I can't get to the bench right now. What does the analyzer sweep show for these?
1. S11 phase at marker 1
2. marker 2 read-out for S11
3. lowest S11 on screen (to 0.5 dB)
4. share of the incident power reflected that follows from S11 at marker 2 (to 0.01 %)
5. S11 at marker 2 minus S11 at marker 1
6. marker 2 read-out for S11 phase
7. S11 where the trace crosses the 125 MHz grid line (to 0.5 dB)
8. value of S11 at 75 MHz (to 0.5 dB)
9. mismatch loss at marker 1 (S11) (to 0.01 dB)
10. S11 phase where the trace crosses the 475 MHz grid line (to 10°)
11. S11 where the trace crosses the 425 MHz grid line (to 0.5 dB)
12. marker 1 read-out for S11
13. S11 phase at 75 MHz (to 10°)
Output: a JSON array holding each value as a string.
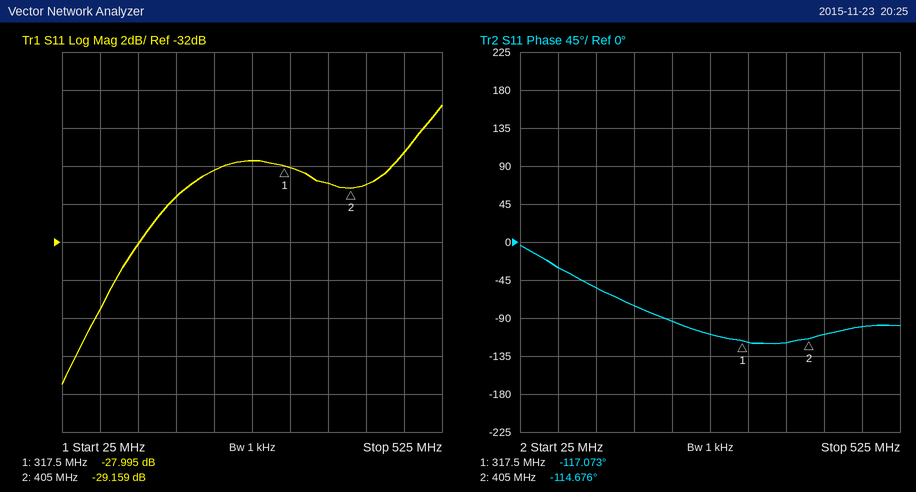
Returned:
["-117.073°", "-29.159 dB", "-39.5 dB", "0.12 %", "-1.164 dB", "-114.676°", "-32.0 dB", "-35.5 dB", "0.01 dB", "-100°", "-29.0 dB", "-27.995 dB", "-30°"]
